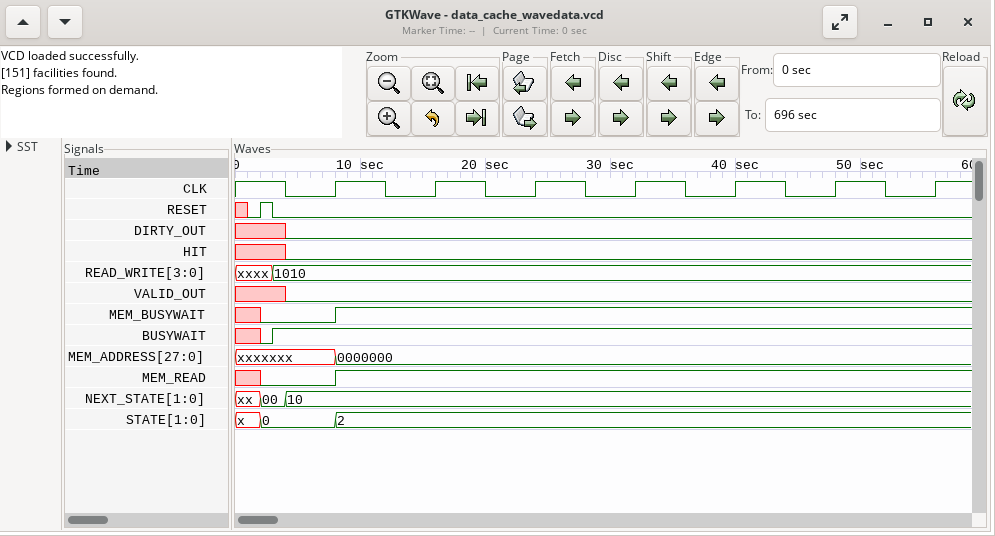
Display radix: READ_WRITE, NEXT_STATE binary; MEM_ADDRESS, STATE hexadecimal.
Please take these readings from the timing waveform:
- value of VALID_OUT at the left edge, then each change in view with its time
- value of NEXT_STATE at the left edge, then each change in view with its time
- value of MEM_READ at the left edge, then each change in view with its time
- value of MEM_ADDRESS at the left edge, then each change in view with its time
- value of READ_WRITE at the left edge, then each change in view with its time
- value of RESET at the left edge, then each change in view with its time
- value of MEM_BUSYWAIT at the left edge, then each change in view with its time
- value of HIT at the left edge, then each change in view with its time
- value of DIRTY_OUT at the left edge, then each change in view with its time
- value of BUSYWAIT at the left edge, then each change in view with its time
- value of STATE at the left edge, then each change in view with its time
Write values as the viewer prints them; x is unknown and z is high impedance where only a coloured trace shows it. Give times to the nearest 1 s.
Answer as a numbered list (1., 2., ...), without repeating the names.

1. x, 0 at 4 s
2. xx, 00 at 2 s, 10 at 4 s
3. x, 0 at 2 s, 1 at 8 s
4. xxxxxxx, 0000000 at 8 s
5. xxxx, 1010 at 3 s
6. x, 0 at 1 s, 1 at 2 s, 0 at 3 s
7. x, 0 at 2 s, 1 at 8 s
8. x, 0 at 4 s
9. x, 0 at 4 s
10. x, 0 at 2 s, 1 at 3 s
11. x, 0 at 2 s, 2 at 8 s
